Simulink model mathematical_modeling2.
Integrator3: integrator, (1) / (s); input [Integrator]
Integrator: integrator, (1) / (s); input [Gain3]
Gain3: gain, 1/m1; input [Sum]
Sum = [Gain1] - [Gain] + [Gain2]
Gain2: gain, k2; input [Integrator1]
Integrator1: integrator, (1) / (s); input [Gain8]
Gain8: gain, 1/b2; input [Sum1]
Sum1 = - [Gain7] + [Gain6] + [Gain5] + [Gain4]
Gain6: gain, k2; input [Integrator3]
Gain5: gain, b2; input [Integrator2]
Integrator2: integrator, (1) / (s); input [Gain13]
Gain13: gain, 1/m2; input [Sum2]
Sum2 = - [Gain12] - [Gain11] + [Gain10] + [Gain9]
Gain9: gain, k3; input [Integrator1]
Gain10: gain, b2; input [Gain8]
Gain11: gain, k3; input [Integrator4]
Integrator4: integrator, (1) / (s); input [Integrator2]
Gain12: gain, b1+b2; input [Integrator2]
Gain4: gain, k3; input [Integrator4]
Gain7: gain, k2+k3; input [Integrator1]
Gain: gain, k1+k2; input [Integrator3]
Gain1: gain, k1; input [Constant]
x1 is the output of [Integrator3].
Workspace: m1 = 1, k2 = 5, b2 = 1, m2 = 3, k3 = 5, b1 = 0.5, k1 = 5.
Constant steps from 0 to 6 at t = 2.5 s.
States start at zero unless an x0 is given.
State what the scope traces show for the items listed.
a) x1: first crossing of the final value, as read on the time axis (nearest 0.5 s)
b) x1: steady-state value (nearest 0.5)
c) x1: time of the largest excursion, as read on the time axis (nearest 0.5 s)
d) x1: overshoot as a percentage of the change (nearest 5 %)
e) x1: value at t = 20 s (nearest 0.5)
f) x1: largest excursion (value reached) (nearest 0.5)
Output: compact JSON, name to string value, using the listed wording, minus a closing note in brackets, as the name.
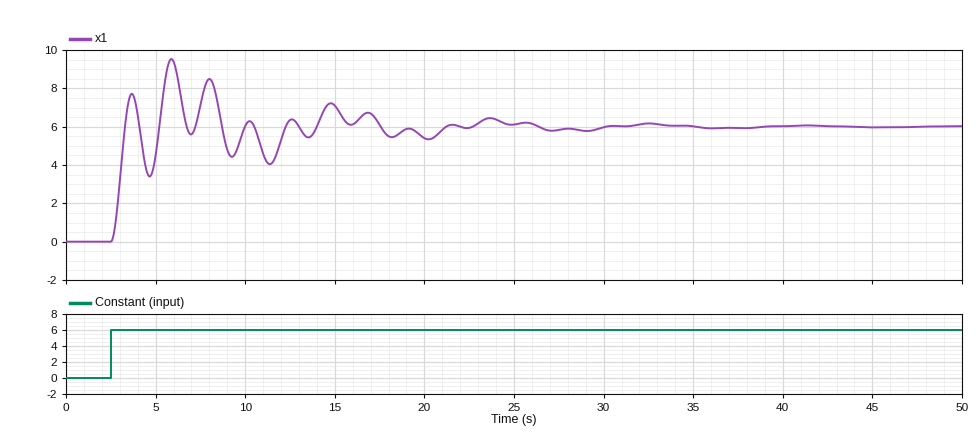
{"x1: first crossing of the final value, as read on the time axis": "3.5 s", "x1: steady-state value": "6.0", "x1: time of the largest excursion, as read on the time axis": "6.0 s", "x1: overshoot as a percentage of the change": "60 %", "x1: value at t = 20 s": "5.5", "x1: largest excursion (value reached)": "9.5"}
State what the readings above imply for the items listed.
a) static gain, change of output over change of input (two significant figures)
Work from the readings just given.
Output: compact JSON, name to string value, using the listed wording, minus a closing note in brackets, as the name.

{"static gain, change of output over change of input": "1.0"}
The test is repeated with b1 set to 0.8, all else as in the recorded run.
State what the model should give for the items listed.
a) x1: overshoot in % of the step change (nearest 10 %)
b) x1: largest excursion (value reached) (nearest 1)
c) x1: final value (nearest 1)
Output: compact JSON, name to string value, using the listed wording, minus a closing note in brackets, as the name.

{"x1: overshoot in % of the step change": "50 %", "x1: largest excursion (value reached)": "9", "x1: final value": "6"}
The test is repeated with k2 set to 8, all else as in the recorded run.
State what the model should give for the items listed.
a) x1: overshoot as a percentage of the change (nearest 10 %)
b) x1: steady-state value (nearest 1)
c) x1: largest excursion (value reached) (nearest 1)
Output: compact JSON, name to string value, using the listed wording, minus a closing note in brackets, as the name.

{"x1: overshoot as a percentage of the change": "50 %", "x1: steady-state value": "6", "x1: largest excursion (value reached)": "9"}
